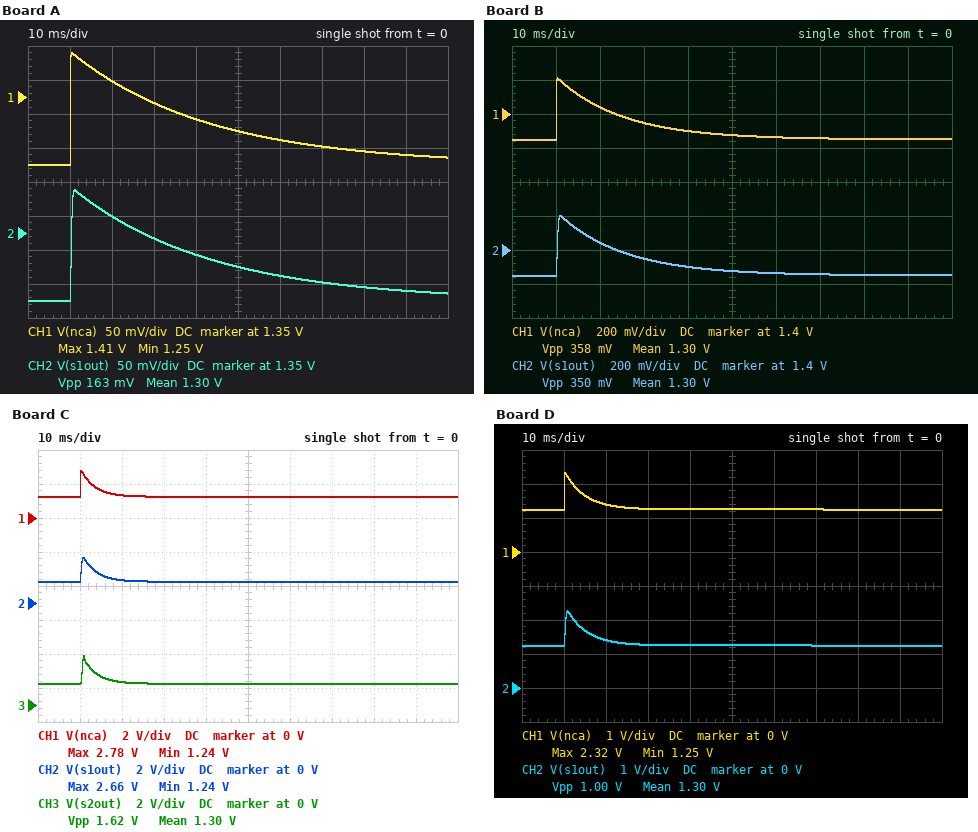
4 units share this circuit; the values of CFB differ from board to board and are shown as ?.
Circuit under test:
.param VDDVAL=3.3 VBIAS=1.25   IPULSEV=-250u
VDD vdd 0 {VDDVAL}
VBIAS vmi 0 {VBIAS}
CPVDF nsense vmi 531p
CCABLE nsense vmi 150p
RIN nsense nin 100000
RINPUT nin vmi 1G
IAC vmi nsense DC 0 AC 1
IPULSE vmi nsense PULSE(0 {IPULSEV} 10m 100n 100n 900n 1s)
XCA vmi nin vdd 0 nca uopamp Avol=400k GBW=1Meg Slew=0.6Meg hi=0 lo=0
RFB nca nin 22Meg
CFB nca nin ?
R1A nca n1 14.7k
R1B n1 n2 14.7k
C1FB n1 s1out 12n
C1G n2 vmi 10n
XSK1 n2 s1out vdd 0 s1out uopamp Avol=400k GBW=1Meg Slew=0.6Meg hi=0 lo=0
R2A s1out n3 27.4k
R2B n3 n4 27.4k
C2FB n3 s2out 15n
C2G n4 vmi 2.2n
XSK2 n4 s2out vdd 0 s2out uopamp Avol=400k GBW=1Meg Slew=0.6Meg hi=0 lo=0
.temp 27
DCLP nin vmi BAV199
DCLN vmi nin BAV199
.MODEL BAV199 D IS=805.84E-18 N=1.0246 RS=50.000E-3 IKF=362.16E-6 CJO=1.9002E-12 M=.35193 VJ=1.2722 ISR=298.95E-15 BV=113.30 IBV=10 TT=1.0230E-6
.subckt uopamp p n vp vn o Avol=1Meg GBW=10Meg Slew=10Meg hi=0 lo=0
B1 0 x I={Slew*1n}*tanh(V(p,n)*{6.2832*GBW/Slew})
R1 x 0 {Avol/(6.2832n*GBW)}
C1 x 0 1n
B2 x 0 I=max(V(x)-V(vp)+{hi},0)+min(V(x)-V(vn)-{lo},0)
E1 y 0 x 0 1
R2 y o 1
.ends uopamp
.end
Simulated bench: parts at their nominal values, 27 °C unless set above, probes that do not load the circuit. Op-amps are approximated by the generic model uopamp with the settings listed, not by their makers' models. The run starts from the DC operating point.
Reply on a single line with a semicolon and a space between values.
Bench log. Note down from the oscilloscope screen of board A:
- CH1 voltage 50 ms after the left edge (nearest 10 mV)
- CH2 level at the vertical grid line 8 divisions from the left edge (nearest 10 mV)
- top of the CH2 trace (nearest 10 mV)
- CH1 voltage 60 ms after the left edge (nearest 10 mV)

1.30 V; 1.27 V; 1.41 V; 1.29 V
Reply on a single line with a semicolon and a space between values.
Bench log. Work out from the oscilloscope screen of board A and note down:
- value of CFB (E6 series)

1.5 nF
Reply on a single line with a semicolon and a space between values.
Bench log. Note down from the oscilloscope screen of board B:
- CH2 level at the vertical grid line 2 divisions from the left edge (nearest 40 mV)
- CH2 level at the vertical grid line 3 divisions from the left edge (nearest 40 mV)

1.44 V; 1.36 V
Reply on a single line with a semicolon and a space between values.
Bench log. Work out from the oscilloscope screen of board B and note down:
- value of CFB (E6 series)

680 pF
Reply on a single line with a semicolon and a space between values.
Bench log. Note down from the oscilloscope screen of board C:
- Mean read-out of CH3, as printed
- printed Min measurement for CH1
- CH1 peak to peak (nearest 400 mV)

1.30 V; 1.24 V; 1.6 V
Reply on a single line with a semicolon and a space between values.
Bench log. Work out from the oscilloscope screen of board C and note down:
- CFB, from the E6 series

150 pF
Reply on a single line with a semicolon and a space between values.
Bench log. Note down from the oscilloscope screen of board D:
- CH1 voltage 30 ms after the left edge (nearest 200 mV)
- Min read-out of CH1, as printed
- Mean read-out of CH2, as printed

1.2 V; 1.25 V; 1.30 V
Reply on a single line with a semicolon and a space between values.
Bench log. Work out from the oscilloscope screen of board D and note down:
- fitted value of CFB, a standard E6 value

220 pF
